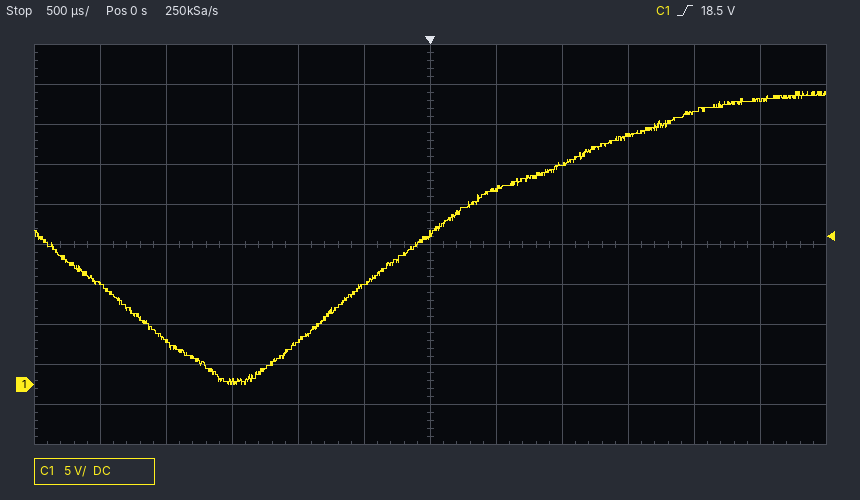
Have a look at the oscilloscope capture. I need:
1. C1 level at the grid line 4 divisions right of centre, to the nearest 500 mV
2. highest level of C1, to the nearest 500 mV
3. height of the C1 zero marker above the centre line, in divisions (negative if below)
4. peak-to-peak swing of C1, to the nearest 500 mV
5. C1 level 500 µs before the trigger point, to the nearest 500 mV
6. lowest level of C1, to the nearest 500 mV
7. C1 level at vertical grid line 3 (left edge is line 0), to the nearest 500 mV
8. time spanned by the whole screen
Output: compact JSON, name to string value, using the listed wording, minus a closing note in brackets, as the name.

{"C1 level at the grid line 4 divisions right of centre, to the nearest 500 mV": "34.0 V", "highest level of C1, to the nearest 500 mV": "36.5 V", "height of the C1 zero marker above the centre line, in divisions": "-3.5 div", "peak-to-peak swing of C1, to the nearest 500 mV": "36.5 V", "C1 level 500 µs before the trigger point, to the nearest 500 mV": "12.5 V", "lowest level of C1, to the nearest 500 mV": "0.0 V", "C1 level at vertical grid line 3 (left edge is line 0), to the nearest 500 mV": "500 mV", "time spanned by the whole screen": "6 ms"}
